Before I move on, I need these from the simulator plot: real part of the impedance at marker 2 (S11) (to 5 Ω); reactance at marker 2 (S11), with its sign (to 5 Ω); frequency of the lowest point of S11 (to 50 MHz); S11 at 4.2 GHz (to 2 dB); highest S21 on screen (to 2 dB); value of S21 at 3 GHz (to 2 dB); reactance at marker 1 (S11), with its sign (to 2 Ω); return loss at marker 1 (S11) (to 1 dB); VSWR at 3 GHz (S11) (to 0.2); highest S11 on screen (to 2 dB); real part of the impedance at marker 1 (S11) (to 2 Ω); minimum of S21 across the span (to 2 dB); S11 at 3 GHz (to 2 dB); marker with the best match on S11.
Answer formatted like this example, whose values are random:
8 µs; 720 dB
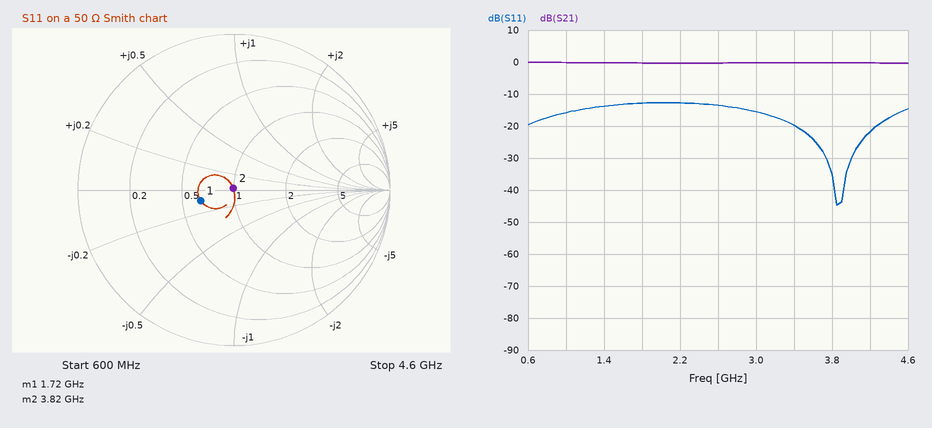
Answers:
50 Ω; 0 Ω; 3.85 GHz; -22 dB; 0 dB; 0 dB; -4 Ω; 13 dB; 1.4; -12 dB; 32 Ω; 0 dB; -16 dB; marker 2
